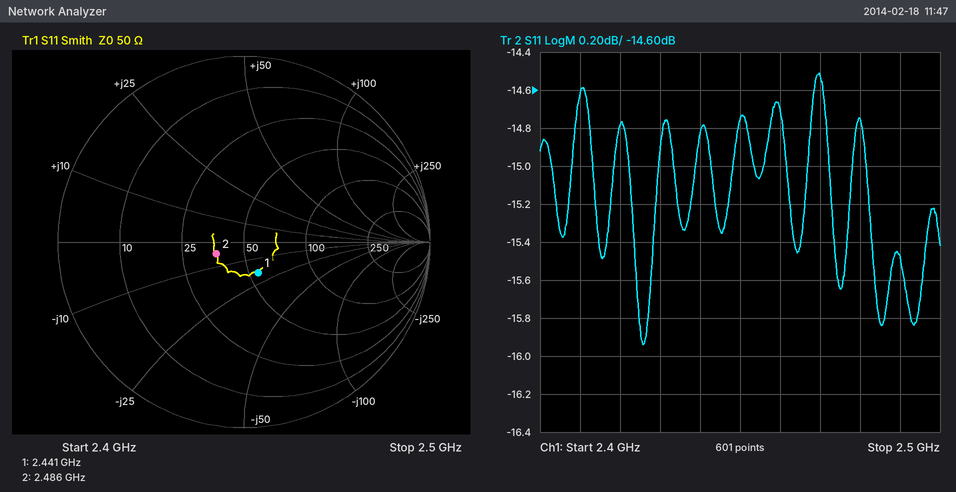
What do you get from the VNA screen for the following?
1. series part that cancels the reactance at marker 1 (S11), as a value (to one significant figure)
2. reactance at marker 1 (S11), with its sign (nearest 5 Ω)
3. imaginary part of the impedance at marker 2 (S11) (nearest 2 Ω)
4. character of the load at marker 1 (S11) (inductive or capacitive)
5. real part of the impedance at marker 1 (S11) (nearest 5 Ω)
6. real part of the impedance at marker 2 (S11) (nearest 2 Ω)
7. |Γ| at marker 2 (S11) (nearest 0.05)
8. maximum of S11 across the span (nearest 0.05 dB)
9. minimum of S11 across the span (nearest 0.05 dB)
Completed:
1 nH
-20 Ω
-4 Ω
capacitive
55 Ω
36 Ω
0.15
-14.50 dB
-15.95 dB
